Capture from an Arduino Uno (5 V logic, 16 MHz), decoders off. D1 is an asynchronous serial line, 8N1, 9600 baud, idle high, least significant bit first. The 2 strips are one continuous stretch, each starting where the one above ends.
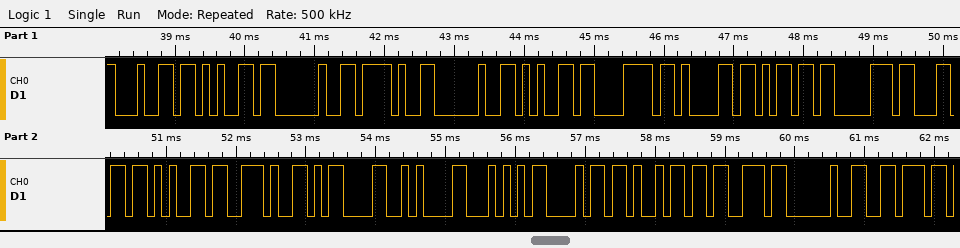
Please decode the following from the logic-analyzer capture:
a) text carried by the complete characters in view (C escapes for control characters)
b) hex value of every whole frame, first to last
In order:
"de / example.\r\nThis v"
64 65 20 2F 20 65 78 61 6D 70 6C 65 2E 0D 0A 54 68 69 73 20 76
